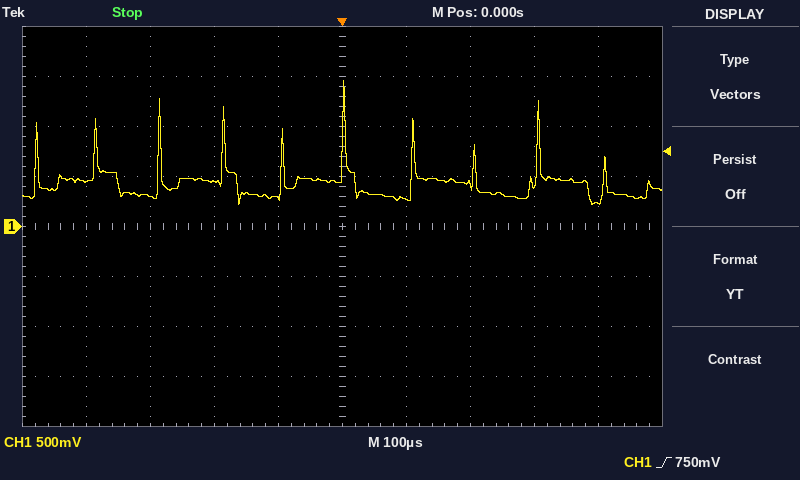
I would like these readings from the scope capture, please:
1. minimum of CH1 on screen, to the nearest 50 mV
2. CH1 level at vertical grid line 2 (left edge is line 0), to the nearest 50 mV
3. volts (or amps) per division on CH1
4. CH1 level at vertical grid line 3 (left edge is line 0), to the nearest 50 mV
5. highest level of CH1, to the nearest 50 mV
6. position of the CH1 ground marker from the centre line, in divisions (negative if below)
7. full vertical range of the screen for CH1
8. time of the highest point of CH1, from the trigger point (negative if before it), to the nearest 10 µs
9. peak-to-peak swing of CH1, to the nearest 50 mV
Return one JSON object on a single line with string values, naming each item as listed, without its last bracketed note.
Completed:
{"minimum of CH1 on screen, to the nearest 50 mV": "200 mV", "CH1 level at vertical grid line 2 (left edge is line 0), to the nearest 50 mV": "300 mV", "volts (or amps) per division on CH1": "500 mV", "CH1 level at vertical grid line 3 (left edge is line 0), to the nearest 50 mV": "450 mV", "highest level of CH1, to the nearest 50 mV": "1.45 V", "position of the CH1 ground marker from the centre line, in divisions": "0.0 div", "full vertical range of the screen for CH1": "4 V", "time of the highest point of CH1, from the trigger point (negative if before it), to the nearest 10 µs": "0 µs", "peak-to-peak swing of CH1, to the nearest 50 mV": "1.25 V"}
